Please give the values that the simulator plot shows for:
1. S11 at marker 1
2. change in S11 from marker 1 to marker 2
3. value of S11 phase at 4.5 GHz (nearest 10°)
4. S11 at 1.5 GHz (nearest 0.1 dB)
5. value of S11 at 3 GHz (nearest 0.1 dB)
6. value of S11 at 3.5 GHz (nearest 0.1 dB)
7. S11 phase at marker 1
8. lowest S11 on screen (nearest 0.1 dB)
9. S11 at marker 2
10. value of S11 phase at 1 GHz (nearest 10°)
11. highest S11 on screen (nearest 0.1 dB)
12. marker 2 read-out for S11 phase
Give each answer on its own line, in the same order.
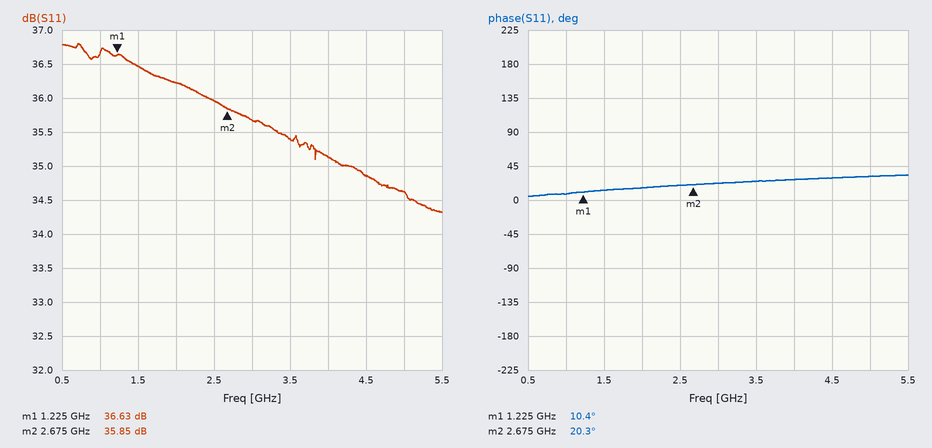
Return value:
36.63 dB
-0.78 dB
30°
36.5 dB
35.7 dB
35.4 dB
10.4°
34.3 dB
35.85 dB
10°
36.8 dB
20.3°
